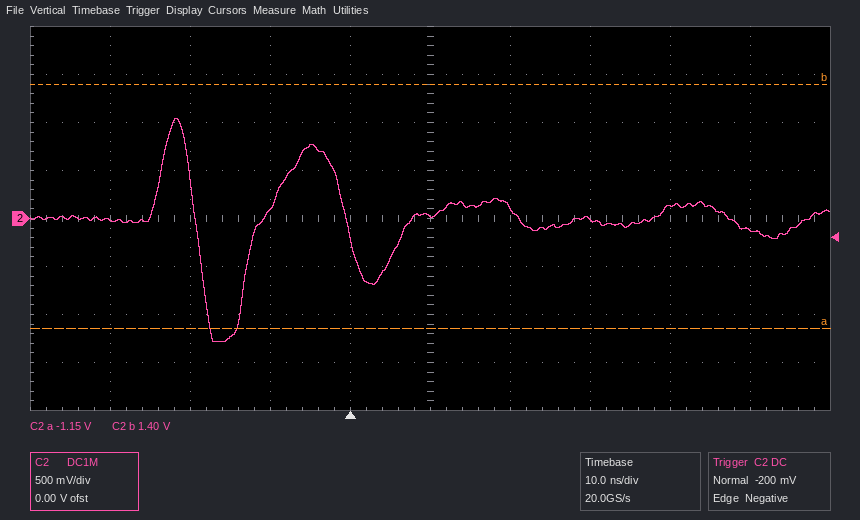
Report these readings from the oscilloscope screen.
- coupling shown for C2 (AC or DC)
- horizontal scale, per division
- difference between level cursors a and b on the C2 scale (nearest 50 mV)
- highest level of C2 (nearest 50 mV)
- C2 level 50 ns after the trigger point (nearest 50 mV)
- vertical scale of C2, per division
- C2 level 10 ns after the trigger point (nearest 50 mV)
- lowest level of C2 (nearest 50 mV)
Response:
DC
10 ns
2.55 V
1.05 V
-100 mV
500 mV
50 mV
-1.30 V
